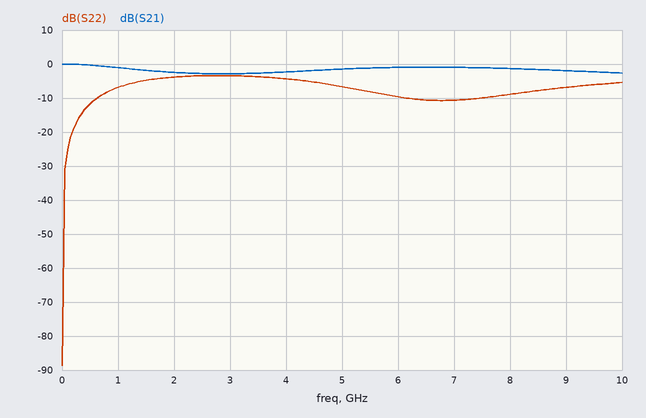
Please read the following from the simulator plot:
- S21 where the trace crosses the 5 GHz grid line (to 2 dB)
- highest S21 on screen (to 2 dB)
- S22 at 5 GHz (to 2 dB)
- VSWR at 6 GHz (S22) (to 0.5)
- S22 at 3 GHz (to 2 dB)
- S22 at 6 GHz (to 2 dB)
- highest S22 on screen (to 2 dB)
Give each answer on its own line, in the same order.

-2 dB
0 dB
-6 dB
2.0
-4 dB
-10 dB
-4 dB
